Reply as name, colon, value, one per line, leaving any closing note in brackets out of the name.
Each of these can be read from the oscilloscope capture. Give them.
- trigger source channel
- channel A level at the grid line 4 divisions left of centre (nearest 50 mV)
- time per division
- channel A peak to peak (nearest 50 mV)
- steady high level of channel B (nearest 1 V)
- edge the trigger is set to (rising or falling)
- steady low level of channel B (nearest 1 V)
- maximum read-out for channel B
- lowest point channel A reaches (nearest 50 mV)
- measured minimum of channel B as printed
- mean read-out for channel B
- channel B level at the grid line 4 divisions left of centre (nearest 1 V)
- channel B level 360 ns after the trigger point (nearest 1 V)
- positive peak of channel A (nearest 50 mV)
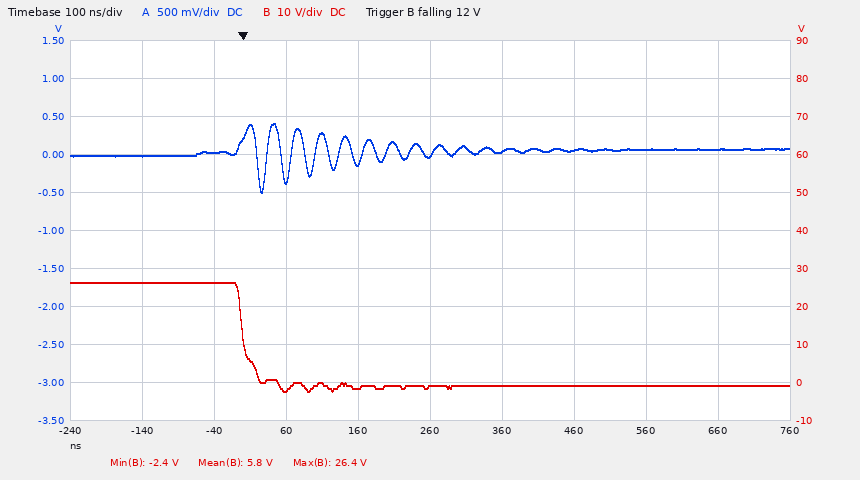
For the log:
trigger source channel: channel B
channel A level at the grid line 4 divisions left of centre: 0 mV
time per division: 100 ns
channel A peak to peak: 900 mV
steady high level of channel B: 26 V
edge the trigger is set to: falling
steady low level of channel B: -1 V
maximum read-out for channel B: 26.4 V
lowest point channel A reaches: -500 mV
measured minimum of channel B as printed: -2.4 V
mean read-out for channel B: 5.8 V
channel B level at the grid line 4 divisions left of centre: 26 V
channel B level 360 ns after the trigger point: -1 V
positive peak of channel A: 400 mV
